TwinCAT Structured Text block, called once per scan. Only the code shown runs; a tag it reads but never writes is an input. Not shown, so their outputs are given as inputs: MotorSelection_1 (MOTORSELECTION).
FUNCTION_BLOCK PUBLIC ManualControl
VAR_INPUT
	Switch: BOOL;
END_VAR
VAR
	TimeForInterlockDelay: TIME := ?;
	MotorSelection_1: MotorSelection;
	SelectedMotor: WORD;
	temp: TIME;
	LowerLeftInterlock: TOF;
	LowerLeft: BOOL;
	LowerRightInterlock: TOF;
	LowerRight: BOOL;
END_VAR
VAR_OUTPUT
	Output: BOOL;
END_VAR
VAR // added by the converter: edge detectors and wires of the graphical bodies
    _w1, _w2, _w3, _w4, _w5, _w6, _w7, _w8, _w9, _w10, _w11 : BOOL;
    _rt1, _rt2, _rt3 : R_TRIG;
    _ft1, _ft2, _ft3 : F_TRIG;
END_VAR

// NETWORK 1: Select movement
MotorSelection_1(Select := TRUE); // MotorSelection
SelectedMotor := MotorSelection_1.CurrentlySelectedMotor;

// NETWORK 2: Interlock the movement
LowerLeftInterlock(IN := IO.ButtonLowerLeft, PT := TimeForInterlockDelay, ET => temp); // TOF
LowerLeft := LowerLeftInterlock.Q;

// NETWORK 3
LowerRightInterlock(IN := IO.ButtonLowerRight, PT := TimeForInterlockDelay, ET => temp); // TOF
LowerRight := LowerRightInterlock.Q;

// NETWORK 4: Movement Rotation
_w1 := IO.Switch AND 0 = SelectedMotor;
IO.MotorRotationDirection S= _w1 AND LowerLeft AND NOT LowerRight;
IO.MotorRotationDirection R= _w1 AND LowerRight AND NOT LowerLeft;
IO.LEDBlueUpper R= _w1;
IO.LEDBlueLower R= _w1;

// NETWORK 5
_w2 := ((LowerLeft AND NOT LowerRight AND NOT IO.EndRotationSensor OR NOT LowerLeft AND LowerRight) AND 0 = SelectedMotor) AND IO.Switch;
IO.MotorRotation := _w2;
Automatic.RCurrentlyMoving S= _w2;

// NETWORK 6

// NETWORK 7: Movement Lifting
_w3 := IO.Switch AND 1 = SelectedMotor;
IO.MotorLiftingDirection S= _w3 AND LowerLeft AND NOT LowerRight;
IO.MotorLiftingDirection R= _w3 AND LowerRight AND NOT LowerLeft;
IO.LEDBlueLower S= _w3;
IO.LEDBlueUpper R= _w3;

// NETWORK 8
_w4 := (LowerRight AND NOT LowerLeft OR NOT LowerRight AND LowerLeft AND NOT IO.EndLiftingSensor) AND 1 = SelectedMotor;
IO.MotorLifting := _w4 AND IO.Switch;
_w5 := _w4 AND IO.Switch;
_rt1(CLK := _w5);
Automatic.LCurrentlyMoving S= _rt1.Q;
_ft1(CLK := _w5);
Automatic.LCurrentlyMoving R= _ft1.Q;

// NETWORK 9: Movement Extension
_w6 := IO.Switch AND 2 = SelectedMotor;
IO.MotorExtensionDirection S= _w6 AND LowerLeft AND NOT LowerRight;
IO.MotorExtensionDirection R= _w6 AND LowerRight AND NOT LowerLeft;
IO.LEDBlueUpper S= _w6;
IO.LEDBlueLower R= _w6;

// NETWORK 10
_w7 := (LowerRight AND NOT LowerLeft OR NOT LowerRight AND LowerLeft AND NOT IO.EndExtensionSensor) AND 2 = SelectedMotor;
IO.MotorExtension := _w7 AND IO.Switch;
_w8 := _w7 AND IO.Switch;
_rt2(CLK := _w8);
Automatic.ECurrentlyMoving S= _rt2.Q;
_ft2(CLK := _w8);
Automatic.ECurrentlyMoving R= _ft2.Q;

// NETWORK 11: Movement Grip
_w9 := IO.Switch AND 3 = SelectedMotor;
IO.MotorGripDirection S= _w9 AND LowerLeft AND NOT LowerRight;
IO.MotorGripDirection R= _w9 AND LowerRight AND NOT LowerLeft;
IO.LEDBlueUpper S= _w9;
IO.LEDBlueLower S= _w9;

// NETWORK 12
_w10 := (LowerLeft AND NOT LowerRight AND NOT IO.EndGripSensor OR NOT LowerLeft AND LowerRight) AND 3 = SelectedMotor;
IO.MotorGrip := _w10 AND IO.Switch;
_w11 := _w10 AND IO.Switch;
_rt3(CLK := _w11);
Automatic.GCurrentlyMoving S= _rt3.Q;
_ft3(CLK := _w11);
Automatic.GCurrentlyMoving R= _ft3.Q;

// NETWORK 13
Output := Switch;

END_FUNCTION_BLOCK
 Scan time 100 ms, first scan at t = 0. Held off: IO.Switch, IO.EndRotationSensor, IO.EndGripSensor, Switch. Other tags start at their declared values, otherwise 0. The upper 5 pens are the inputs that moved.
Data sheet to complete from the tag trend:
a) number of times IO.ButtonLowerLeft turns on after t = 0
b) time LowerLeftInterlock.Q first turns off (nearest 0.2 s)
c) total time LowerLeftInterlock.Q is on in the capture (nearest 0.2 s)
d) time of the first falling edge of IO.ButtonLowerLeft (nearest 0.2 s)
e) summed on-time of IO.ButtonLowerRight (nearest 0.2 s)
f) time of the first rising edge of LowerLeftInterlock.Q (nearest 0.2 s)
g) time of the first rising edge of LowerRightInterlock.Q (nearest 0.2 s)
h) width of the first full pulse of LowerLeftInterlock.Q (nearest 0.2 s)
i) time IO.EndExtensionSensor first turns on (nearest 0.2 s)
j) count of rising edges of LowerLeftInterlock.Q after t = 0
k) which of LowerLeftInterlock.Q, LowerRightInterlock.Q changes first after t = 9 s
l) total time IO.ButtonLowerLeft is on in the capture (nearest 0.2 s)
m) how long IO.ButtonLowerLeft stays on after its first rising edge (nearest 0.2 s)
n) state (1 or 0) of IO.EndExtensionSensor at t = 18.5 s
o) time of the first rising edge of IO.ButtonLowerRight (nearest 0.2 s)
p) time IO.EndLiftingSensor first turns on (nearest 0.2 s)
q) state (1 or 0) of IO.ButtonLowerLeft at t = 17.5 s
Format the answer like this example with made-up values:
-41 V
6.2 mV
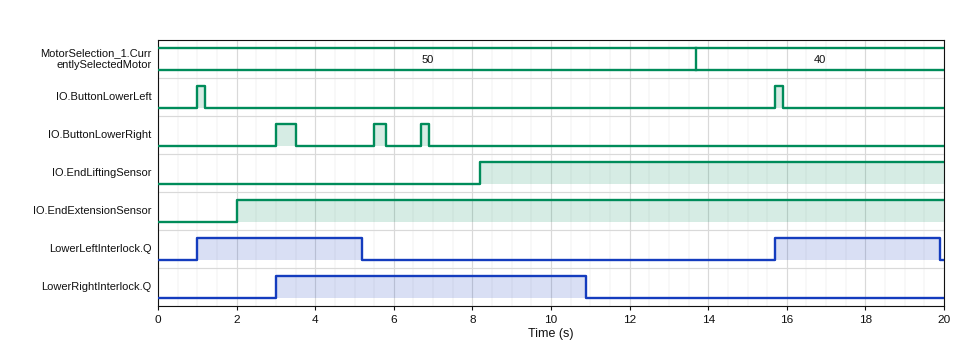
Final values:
2
5.2 s
8.4 s
1.2 s
1.0 s
1.0 s
3.0 s
4.2 s
2.0 s
2
LowerRightInterlock.Q
0.4 s
0.2 s
1
3.0 s
8.2 s
0
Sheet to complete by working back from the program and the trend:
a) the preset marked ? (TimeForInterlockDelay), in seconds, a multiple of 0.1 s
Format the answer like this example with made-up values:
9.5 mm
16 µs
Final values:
4.0 s
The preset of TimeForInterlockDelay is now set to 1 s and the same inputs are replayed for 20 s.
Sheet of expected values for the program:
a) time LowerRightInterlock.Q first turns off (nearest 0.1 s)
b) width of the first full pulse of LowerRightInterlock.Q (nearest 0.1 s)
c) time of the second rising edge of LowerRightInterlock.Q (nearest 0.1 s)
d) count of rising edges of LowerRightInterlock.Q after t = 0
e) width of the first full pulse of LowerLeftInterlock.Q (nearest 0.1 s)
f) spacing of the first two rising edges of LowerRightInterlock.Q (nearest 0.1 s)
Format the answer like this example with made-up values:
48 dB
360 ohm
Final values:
4.5 s
1.5 s
5.5 s
2
1.2 s
2.5 s
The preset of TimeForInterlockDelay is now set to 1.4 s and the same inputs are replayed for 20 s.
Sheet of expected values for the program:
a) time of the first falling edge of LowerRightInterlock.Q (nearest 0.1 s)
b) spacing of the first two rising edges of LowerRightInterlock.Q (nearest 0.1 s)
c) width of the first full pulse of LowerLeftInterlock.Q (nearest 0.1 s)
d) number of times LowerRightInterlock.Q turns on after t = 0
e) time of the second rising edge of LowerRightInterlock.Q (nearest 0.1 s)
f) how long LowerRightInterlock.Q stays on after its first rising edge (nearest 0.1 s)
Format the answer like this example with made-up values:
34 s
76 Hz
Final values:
4.9 s
2.5 s
1.6 s
2
5.5 s
1.9 s
